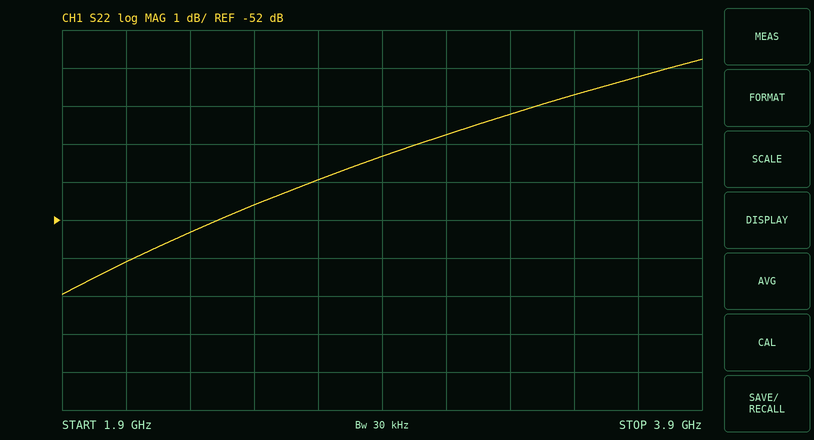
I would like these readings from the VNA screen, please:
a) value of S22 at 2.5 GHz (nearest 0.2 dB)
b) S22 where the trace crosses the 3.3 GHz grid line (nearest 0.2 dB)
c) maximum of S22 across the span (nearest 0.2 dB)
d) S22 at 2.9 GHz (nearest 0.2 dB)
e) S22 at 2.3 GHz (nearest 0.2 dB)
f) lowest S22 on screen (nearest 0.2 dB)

-51.6 dB
-49.2 dB
-47.8 dB
-50.4 dB
-52.4 dB
-54.0 dB
